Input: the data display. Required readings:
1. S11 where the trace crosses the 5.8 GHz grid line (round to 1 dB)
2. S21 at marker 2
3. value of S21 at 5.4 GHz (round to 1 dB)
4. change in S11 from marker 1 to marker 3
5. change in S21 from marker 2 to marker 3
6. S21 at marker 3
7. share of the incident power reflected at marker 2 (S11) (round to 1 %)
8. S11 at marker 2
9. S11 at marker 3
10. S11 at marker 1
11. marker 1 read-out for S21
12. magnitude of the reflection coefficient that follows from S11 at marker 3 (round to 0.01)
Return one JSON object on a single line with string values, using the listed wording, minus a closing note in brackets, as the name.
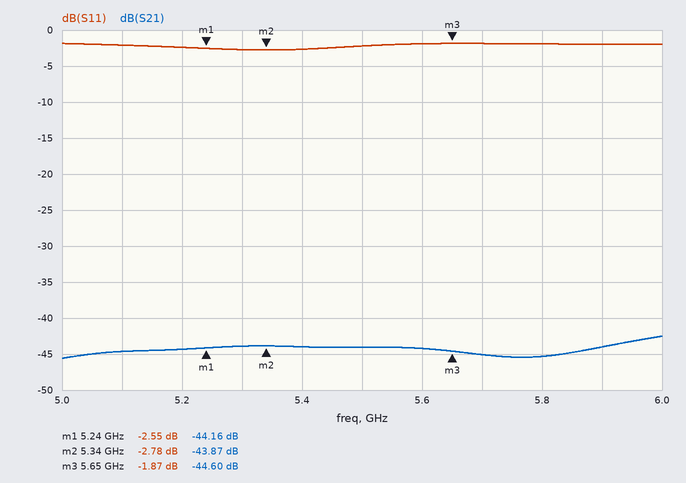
{"S11 where the trace crosses the 5.8 GHz grid line": "-2 dB", "S21 at marker 2": "-43.87 dB", "value of S21 at 5.4 GHz": "-44 dB", "change in S11 from marker 1 to marker 3": "0.68 dB", "change in S21 from marker 2 to marker 3": "-0.73 dB", "S21 at marker 3": "-44.60 dB", "share of the incident power reflected at marker 2 (S11)": "53 %", "S11 at marker 2": "-2.78 dB", "S11 at marker 3": "-1.87 dB", "S11 at marker 1": "-2.55 dB", "marker 1 read-out for S21": "-44.16 dB", "magnitude of the reflection coefficient that follows from S11 at marker 3": "0.81"}
